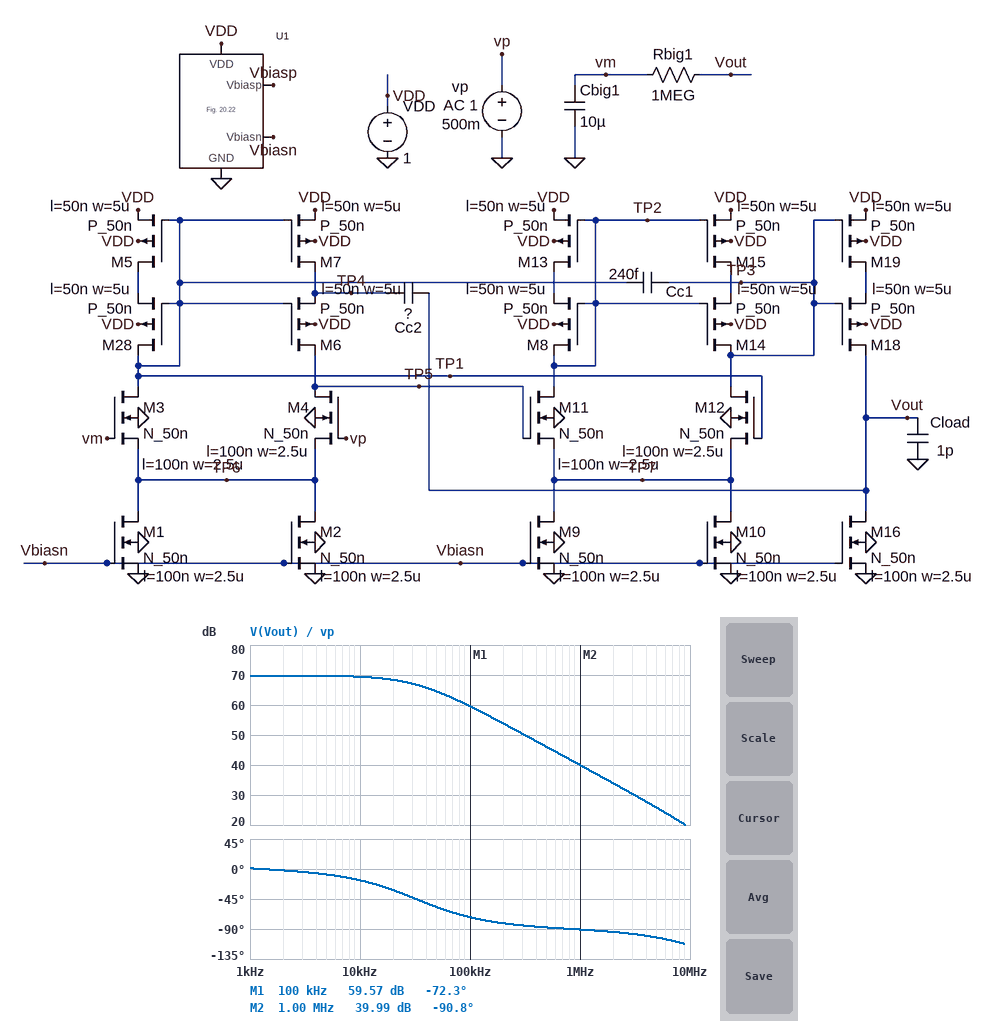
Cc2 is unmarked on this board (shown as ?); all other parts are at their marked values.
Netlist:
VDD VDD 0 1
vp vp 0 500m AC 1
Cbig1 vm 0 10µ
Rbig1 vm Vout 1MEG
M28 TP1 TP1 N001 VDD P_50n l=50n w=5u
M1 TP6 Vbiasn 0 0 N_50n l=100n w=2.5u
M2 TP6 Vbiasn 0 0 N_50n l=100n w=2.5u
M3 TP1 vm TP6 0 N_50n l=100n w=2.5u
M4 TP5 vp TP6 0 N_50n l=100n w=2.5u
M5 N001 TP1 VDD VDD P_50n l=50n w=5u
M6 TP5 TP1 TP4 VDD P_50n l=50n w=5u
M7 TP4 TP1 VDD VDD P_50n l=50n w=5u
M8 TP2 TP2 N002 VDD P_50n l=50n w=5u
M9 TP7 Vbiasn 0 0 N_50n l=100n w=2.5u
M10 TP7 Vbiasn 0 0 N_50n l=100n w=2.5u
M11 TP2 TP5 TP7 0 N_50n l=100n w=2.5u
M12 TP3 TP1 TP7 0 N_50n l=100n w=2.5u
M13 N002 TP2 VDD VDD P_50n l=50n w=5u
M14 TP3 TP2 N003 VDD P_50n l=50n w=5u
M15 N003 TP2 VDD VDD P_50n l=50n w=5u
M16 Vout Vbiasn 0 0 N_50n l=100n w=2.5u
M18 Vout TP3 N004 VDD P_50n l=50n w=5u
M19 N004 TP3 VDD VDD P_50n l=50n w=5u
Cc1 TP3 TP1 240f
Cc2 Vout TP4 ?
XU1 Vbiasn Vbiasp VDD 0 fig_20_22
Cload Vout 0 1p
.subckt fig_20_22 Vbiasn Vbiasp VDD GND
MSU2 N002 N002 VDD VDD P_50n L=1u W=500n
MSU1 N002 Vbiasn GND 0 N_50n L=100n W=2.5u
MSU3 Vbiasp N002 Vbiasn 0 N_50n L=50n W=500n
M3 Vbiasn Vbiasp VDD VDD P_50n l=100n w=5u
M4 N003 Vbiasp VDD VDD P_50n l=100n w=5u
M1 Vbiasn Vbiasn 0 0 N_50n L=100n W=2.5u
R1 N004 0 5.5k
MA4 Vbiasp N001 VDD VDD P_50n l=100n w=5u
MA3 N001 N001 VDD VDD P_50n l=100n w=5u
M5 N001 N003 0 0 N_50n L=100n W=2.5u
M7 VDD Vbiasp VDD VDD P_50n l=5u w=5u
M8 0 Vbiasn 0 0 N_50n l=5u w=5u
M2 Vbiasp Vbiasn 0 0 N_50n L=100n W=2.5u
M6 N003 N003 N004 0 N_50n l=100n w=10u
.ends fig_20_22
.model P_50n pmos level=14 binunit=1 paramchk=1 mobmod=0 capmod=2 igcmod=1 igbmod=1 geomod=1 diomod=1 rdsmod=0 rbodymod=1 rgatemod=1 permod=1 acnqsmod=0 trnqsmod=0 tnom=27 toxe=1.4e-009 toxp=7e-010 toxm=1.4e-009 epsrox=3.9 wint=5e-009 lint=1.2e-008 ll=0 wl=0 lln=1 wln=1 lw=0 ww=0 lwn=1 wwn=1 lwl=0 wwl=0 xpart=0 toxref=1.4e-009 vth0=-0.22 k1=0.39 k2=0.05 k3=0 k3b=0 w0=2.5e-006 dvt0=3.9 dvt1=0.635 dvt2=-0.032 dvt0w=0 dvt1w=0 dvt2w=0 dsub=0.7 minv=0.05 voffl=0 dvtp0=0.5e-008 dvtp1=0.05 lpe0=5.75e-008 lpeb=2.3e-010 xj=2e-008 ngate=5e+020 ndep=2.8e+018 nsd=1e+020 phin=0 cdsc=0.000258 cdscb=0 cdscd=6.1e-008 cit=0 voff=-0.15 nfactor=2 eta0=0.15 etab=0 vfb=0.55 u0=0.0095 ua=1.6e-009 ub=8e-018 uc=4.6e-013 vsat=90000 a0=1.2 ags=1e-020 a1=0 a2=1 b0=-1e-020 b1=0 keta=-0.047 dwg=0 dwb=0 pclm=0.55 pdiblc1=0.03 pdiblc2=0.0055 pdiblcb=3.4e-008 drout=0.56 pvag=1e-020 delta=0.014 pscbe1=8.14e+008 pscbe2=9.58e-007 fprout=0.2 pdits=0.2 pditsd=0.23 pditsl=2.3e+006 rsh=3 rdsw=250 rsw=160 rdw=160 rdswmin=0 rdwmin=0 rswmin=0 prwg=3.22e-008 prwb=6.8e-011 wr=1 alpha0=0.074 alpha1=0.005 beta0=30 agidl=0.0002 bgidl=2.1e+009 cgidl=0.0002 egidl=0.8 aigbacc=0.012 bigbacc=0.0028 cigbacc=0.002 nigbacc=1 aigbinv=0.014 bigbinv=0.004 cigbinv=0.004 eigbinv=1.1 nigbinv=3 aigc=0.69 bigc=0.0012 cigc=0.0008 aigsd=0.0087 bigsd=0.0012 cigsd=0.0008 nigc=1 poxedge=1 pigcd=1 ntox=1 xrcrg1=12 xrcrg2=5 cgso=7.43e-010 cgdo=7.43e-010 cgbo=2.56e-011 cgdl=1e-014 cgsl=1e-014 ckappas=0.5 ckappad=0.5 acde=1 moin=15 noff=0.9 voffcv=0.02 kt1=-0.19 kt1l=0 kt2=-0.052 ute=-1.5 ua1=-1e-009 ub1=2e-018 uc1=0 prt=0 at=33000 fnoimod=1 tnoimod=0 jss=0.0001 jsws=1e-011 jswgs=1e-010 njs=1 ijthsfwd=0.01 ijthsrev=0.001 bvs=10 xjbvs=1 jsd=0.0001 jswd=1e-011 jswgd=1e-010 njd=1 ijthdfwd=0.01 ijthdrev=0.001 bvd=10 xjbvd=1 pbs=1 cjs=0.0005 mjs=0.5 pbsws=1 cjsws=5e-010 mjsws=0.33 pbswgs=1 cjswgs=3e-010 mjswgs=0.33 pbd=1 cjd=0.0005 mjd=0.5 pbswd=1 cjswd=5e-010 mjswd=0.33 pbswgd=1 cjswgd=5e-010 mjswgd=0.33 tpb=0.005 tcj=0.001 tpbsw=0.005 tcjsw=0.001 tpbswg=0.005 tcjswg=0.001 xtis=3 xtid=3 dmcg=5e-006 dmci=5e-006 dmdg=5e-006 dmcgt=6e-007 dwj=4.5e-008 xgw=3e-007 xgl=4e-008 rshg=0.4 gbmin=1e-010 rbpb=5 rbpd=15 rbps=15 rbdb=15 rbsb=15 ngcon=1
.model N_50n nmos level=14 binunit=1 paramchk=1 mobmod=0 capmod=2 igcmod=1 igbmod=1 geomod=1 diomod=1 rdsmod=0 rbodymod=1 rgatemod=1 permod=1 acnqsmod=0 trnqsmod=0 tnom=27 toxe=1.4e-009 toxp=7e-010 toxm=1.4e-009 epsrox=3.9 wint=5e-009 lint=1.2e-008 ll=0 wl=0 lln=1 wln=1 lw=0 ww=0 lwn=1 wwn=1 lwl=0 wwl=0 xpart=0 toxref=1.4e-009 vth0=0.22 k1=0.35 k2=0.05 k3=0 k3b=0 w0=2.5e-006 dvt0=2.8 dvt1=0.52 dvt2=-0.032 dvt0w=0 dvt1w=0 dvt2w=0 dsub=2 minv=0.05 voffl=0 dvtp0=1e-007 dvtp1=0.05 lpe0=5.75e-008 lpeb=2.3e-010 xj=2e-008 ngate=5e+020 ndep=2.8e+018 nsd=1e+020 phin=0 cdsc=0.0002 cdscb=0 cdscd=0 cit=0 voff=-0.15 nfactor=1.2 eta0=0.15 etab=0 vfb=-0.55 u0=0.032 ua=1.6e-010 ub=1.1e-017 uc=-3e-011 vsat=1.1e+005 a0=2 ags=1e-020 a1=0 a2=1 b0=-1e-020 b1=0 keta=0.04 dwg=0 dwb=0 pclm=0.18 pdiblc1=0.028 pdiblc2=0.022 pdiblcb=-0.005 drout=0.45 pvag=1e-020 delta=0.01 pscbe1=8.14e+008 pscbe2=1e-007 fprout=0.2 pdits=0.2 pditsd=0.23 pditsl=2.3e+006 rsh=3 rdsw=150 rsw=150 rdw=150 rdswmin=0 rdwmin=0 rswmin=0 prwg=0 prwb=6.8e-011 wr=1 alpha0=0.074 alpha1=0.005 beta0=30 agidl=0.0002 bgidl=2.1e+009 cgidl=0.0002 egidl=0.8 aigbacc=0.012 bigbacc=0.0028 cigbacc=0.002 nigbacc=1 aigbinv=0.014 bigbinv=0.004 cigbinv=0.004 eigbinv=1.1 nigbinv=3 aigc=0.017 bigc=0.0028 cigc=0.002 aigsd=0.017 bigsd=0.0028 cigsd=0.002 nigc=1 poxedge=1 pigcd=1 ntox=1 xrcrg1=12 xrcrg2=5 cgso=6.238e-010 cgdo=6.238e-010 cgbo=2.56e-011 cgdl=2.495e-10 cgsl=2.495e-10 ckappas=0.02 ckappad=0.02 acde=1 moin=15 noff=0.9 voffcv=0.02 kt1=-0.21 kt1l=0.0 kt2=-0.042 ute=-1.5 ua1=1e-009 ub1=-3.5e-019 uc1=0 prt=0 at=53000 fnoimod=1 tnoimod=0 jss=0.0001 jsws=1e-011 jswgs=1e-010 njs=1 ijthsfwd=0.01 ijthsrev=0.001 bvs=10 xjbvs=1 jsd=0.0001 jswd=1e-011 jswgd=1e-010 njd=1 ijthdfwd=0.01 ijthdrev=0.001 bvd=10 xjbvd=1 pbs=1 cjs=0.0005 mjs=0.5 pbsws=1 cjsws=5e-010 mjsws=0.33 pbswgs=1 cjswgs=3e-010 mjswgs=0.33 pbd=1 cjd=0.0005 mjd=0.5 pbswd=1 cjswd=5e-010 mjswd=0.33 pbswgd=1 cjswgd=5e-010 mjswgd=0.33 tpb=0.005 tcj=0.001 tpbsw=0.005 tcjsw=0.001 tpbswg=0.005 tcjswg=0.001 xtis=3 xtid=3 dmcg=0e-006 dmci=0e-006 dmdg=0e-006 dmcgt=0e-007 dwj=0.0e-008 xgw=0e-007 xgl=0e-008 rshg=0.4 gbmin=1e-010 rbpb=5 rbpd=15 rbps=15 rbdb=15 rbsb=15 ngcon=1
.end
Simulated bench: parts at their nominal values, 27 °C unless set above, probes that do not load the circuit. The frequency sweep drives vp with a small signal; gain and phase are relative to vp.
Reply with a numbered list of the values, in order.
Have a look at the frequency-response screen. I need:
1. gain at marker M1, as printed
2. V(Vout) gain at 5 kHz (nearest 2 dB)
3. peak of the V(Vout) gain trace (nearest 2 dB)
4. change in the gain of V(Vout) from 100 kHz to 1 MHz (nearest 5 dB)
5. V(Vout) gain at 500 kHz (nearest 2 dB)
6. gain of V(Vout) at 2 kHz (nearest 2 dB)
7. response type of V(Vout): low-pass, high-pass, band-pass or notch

1. 59.57 dB
2. 70 dB
3. 70 dB
4. -20 dB
5. 46 dB
6. 70 dB
7. low-pass
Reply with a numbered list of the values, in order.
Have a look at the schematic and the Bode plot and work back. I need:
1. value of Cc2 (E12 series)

1. 390 fF
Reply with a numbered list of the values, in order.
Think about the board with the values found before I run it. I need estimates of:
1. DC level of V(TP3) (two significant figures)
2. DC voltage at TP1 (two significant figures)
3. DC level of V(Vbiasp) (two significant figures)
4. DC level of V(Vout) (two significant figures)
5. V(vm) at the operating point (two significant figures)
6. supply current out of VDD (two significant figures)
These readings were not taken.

1. 670 mV
2. 680 mV
3. 650 mV
4. 500 mV
5. 500 mV
6. 96 µA
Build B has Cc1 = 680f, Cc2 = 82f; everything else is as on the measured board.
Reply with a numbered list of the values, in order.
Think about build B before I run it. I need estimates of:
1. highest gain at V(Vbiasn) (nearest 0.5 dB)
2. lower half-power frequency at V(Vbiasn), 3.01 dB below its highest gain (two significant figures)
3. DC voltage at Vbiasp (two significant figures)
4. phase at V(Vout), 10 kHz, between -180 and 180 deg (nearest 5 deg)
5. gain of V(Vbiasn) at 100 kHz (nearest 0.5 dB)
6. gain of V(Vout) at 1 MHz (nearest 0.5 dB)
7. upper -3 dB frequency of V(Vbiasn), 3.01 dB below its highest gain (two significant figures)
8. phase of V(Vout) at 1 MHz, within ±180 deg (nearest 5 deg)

1. -29.5 dB
2. 77 kHz
3. 650 mV
4. -5 deg
5. -31.5 dB
6. 47.5 dB
7. 3.6 MHz
8. -100 deg
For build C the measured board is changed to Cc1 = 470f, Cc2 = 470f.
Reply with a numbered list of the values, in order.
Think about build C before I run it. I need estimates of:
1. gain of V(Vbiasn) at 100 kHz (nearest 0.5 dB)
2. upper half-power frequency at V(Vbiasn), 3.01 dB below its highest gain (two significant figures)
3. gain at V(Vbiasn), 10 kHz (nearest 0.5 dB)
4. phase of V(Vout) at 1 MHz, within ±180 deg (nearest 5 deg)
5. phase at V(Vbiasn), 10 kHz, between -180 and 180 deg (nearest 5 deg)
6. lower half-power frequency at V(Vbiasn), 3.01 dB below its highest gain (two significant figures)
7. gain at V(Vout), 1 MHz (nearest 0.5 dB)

1. -39.5 dB
2. 9.7 MHz
3. -46.0 dB
4. -95 deg
5. 30 deg
6. 23 kHz
7. 38.0 dB
